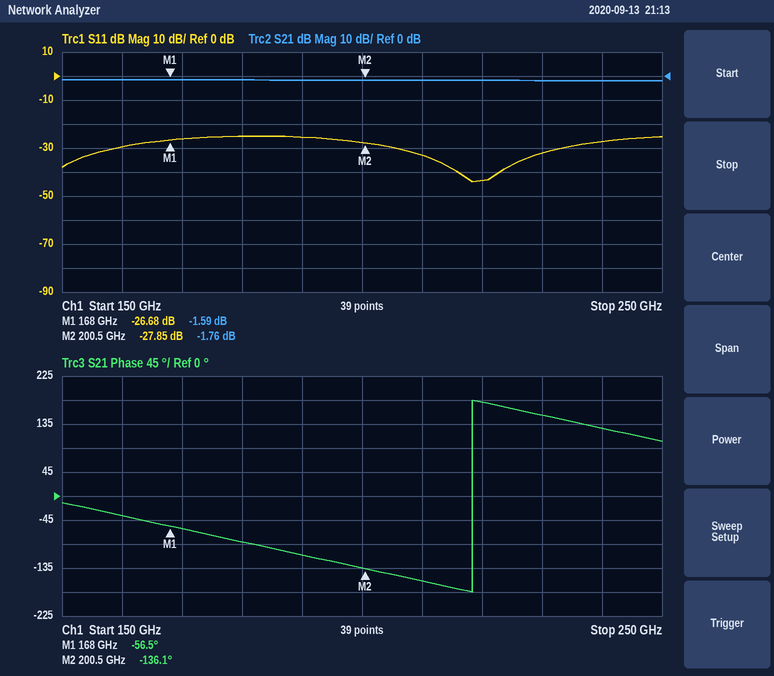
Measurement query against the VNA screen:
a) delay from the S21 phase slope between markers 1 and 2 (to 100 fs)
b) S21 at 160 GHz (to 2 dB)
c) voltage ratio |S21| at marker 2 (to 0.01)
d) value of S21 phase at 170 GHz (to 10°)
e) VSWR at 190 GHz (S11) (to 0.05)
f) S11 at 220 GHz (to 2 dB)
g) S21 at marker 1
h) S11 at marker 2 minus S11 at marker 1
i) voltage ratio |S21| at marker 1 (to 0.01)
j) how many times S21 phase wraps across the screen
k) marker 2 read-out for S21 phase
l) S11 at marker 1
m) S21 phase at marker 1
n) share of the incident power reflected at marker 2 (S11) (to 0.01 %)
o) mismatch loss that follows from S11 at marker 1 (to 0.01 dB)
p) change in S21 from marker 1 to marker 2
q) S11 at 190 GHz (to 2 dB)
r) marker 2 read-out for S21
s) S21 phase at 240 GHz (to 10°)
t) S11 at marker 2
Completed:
6.8 ps
-2 dB
0.82
-60°
1.10
-44 dB
-1.59 dB
-1.17 dB
0.83
1
-136.1°
-26.68 dB
-56.5°
0.16 %
0.01 dB
-0.17 dB
-26 dB
-1.76 dB
130°
-27.85 dB
